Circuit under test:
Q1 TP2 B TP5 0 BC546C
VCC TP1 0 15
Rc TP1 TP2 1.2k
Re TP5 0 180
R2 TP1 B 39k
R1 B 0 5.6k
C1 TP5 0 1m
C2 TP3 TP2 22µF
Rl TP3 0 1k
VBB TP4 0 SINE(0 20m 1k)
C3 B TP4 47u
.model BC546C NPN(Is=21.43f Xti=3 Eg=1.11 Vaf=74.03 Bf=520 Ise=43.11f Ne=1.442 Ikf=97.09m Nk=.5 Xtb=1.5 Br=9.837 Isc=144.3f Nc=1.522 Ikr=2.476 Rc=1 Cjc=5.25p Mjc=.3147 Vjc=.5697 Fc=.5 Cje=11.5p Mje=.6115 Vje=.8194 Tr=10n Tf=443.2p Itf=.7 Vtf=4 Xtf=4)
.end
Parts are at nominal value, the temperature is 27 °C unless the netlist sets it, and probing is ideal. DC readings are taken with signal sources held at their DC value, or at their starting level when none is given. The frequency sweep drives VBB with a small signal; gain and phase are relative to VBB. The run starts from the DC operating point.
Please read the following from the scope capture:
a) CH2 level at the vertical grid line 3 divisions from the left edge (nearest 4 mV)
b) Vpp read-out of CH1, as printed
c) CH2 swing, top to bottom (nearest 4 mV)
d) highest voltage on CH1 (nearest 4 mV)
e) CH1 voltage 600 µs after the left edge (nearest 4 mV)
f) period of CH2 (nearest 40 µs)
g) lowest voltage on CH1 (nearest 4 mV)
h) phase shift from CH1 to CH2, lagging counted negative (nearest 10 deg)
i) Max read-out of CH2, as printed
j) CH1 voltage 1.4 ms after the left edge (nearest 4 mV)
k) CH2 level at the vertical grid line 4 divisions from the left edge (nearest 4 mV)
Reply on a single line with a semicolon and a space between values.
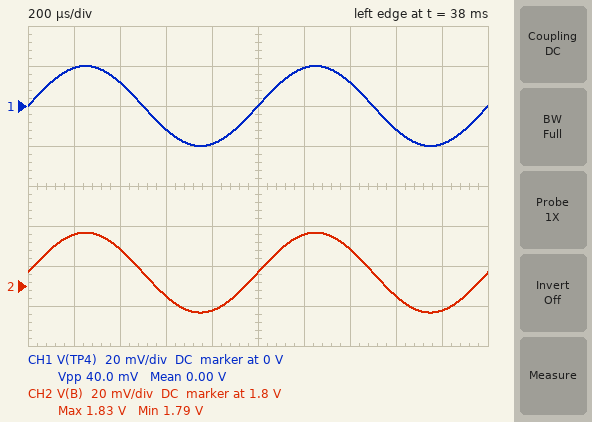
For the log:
1.796 V; 40.0 mV; 40 mV; 20 mV; -12 mV; 1.00 ms; -20 mV; 0 deg; 1.83 V; 12 mV; 1.788 V
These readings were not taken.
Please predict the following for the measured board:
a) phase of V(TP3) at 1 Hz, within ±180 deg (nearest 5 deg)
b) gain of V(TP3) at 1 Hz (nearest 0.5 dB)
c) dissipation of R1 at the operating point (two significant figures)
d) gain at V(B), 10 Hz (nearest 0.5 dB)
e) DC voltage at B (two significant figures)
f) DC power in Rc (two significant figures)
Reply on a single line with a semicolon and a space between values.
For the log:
-25 deg; 0 dB; 580 µW; -0.5 dB; 1.8 V; 47 mW
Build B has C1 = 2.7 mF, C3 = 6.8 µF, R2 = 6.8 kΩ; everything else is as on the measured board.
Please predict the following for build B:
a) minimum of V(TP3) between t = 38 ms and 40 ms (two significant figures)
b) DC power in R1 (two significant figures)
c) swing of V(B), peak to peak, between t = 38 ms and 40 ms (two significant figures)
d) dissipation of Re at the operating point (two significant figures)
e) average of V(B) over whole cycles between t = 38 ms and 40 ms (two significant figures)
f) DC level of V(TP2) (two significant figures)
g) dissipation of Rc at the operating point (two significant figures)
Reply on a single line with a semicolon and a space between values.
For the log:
-6.6 mV; 1.5 mW; 18 mV; 26 mW; 2.9 V; 2.2 V; 140 mW
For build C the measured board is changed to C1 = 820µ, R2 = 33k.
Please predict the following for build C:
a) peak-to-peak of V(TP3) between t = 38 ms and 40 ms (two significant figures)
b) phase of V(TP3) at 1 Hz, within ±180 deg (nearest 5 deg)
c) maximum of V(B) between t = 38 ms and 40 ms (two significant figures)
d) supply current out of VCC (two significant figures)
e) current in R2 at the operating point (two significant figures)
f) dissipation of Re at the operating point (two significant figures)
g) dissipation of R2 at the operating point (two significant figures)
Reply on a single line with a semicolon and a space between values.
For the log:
5.5 V; -30 deg; 2.1 V; 8.1 mA; 390 µA; 11 mW; 5.1 mW
